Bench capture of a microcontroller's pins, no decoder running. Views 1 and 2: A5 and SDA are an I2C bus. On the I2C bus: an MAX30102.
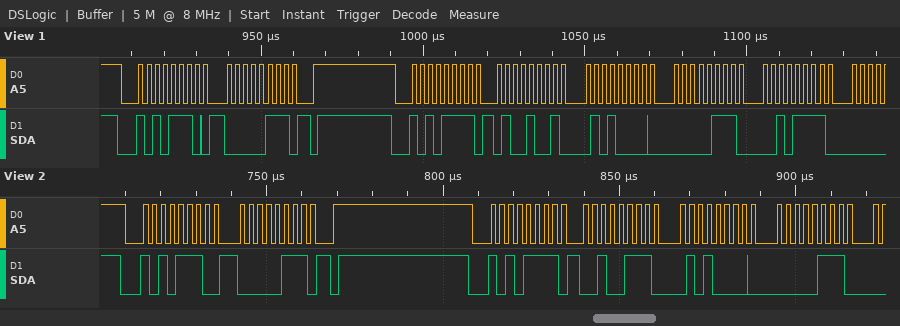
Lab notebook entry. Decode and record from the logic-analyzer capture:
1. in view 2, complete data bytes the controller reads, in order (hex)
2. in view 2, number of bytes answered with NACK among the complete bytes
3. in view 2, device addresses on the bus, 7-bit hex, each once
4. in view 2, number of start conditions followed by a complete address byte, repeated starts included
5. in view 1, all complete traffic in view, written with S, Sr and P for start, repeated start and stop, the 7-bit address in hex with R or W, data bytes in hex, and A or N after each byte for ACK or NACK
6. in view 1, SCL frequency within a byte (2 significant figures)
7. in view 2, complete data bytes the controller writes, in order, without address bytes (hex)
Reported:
27 50 07
0
0x57
2
S 57W A 07 A P S 57R A 49 A 50 A 07 A 2F A
400 kHz
07
